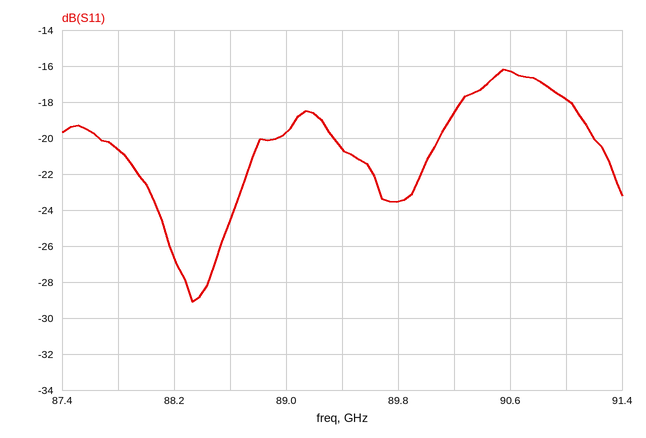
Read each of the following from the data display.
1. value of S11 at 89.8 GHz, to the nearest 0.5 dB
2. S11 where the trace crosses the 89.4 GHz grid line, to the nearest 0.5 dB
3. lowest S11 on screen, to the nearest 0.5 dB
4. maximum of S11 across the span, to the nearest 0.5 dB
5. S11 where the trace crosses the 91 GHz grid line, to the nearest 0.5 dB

-23.5 dB
-20.5 dB
-29.0 dB
-16.0 dB
-18.0 dB
